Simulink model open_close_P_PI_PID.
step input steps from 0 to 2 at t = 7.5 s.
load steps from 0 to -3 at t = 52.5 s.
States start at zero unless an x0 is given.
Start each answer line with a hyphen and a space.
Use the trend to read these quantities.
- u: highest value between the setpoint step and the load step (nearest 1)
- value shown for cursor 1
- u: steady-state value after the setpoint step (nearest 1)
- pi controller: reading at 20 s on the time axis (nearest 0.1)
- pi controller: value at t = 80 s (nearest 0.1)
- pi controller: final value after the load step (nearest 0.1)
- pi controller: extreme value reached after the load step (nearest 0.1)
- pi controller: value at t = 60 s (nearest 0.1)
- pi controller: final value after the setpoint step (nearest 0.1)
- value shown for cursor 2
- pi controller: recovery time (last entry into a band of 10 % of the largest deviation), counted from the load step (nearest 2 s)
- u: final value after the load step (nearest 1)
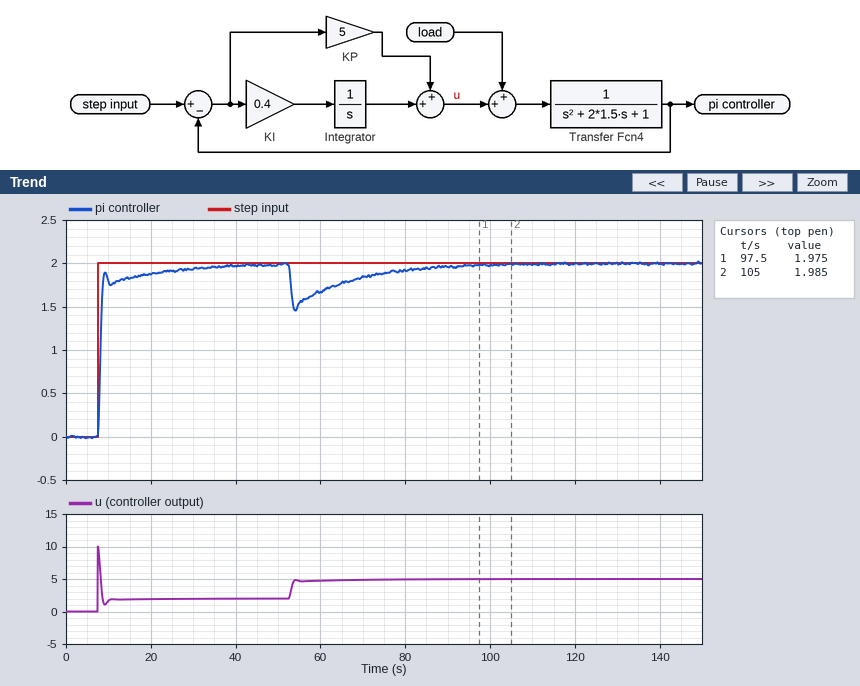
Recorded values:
- 10
- 1.975
- 2
- 1.9
- 1.9
- 2.0
- 1.5
- 1.7
- 2.0
- 1.985
- 34 s
- 5
